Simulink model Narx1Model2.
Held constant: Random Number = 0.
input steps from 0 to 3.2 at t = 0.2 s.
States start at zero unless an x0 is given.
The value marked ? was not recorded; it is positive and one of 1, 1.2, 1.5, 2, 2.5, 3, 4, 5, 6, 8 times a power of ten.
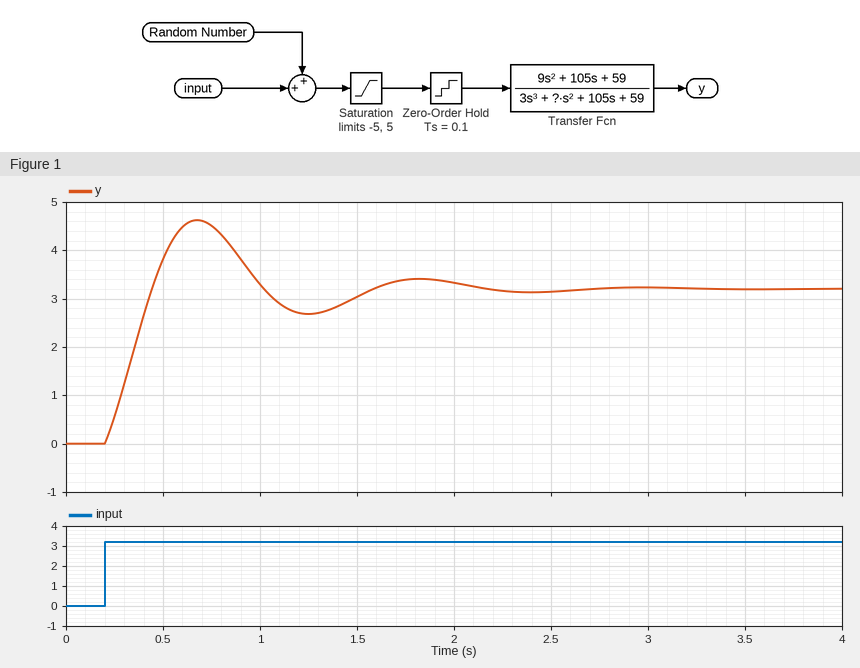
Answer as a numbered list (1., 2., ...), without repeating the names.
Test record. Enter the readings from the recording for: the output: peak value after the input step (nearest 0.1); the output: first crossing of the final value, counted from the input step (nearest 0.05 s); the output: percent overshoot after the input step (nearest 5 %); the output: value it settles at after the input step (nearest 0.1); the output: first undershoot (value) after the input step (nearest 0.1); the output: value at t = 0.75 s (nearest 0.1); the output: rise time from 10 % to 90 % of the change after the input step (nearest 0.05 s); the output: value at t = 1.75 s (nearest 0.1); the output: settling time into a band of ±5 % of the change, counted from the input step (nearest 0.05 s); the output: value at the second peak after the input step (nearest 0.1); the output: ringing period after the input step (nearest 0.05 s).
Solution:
1. 4.6
2. 0.25 s
3. 45 %
4. 3.2
5. 2.7
6. 4.5
7. 0.20 s
8. 3.4
9. 1.75 s
10. 3.4
11. 1.15 s
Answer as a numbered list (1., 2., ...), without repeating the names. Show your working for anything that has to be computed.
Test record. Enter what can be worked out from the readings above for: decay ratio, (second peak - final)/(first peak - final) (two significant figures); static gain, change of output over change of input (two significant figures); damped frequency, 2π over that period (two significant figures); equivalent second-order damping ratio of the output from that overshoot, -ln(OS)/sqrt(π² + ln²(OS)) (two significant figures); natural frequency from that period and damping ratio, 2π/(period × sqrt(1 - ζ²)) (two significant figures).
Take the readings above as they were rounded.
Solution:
1. (3.4 - 3.2) / (4.6 - 3.2) = 0.14
2. (3.2 - 0) / (3.2 - 0) = 1.0
3. 2π / 1.15 = 5.5 rad/s
4. ln(0.45) = -0.799; 0.799 / sqrt(9.870 + 0.638) = 0.25
5. 2π / (1.15 × sqrt(1 - 0.25²)) = 5.6 rad/s
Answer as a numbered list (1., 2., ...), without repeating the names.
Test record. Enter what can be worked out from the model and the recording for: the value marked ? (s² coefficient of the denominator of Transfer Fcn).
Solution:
1. 12
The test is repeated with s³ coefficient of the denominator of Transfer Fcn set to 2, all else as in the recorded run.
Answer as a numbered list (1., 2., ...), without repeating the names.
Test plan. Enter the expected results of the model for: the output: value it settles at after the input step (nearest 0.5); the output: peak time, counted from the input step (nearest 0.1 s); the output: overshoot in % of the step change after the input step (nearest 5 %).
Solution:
1. 3.0
2. 0.4 s
3. 35 %
